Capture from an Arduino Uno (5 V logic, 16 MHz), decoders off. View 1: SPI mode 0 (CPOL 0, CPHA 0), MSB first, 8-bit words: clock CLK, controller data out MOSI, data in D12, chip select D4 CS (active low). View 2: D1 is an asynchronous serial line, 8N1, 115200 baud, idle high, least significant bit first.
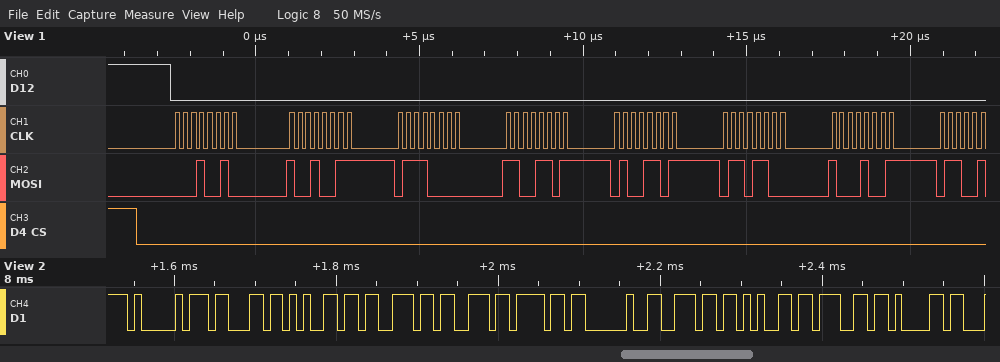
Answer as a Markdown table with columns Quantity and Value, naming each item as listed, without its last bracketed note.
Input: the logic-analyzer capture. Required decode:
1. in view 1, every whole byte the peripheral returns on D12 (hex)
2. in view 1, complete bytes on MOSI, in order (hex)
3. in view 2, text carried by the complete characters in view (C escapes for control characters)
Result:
| Quantity | Value |
|---|---|
| in view 1, every whole byte the peripheral returns on D12 | 00 00 00 00 00 00 00 |
| in view 1, complete bytes on MOSI, in order | 12 93 70 CD 4D 6C 89 |
| in view 2, text carried by the complete characters in view | "Acesso nega" |
